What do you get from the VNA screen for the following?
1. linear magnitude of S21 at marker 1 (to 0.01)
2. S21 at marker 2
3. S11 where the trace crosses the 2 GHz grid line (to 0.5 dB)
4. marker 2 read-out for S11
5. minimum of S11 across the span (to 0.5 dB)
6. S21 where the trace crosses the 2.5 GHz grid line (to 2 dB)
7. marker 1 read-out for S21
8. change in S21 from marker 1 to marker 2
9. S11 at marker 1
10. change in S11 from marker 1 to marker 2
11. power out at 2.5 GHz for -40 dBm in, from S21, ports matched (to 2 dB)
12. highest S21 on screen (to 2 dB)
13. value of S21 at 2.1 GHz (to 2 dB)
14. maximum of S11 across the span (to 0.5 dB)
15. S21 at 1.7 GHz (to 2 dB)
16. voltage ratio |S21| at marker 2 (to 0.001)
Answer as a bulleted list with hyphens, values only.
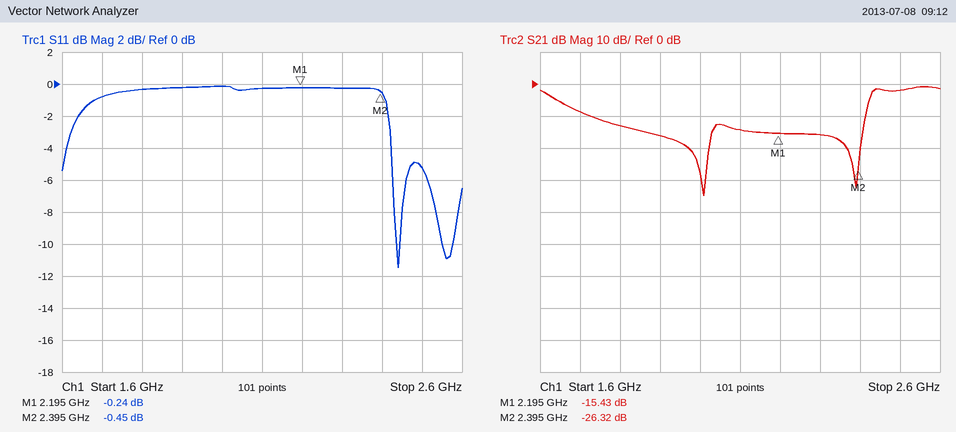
- 0.17
- -26.32 dB
- 0.0 dB
- -0.45 dB
- -11.5 dB
- -2 dB
- -15.43 dB
- -10.89 dB
- -0.24 dB
- -0.21 dB
- -42 dBm
- 0 dB
- -14 dB
- 0.0 dB
- -8 dB
- 0.048
